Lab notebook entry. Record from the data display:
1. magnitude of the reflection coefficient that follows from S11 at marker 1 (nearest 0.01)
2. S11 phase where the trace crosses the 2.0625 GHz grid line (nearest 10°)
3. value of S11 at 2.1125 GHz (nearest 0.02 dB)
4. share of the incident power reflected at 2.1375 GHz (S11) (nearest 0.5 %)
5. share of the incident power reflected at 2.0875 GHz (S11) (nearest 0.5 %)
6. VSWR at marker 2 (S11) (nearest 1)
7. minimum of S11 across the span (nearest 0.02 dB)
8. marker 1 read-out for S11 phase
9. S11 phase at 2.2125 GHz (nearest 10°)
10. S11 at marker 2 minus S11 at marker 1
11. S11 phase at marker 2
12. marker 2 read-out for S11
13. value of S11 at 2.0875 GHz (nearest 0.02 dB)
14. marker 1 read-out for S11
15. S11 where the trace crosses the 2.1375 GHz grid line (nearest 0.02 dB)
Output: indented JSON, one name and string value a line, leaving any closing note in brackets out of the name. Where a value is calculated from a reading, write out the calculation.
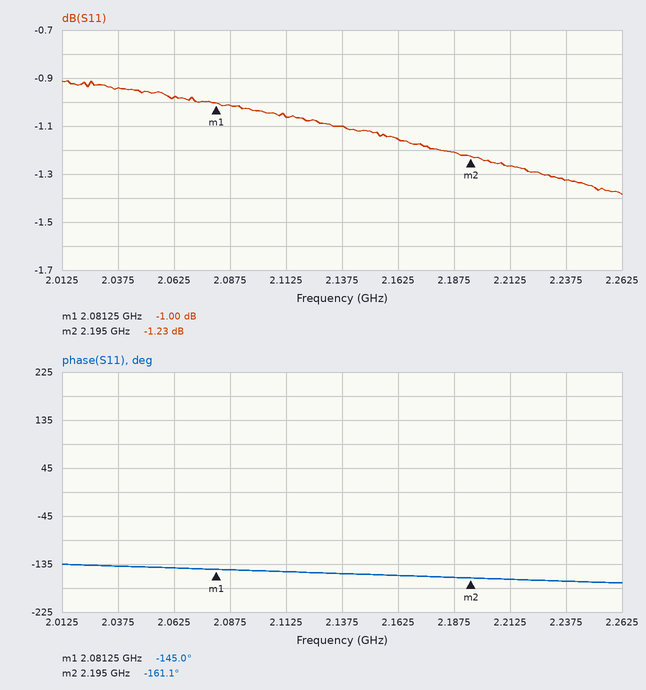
{
  "magnitude of the reflection coefficient that follows from S11 at marker 1": "10^(-1/20) ≈ 0.89",
  "S11 phase where the trace crosses the 2.0625 GHz grid line": "-140°",
  "value of S11 at 2.1125 GHz": "-1.06 dB",
  "share of the incident power reflected at 2.1375 GHz (S11)": "10^(-1.1/10) ≈ 77.6 %, so 77.5 % to the nearest 0.5 %",
  "share of the incident power reflected at 2.0875 GHz (S11)": "10^(-1.02/10) ≈ 79.1 %, so 79.0 % to the nearest 0.5 %",
  "VSWR at marker 2 (S11)": "(1 + 0.8680)/(1 − 0.8680) ≈ 14",
  "minimum of S11 across the span": "-1.38 dB",
  "marker 1 read-out for S11 phase": "-145.0°",
  "S11 phase at 2.2125 GHz": "-160°",
  "S11 at marker 2 minus S11 at marker 1": "-1.23 − (-1) = -0.23 dB",
  "S11 phase at marker 2": "-161.1°",
  "marker 2 read-out for S11": "-1.23 dB",
  "value of S11 at 2.0875 GHz": "-1.02 dB",
  "marker 1 read-out for S11": "-1.00 dB",
  "S11 where the trace crosses the 2.1375 GHz grid line": "-1.10 dB"
}
